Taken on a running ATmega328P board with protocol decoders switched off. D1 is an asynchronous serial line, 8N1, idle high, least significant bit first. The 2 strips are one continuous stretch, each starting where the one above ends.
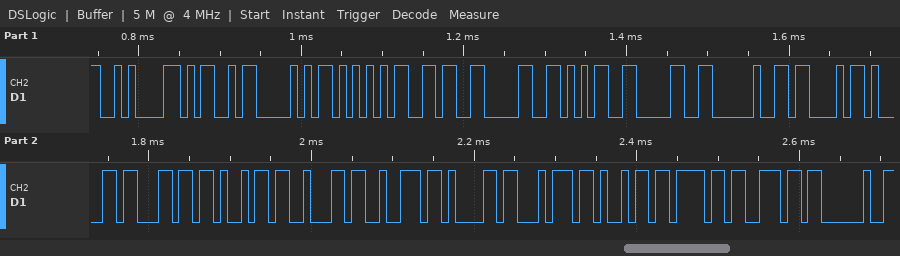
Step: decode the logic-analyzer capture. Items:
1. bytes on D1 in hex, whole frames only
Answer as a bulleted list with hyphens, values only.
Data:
- 0A 4D 50 55 36 30 35 30 20 43 61 6C 69 62 72 61 74 69 6F 6E 20
